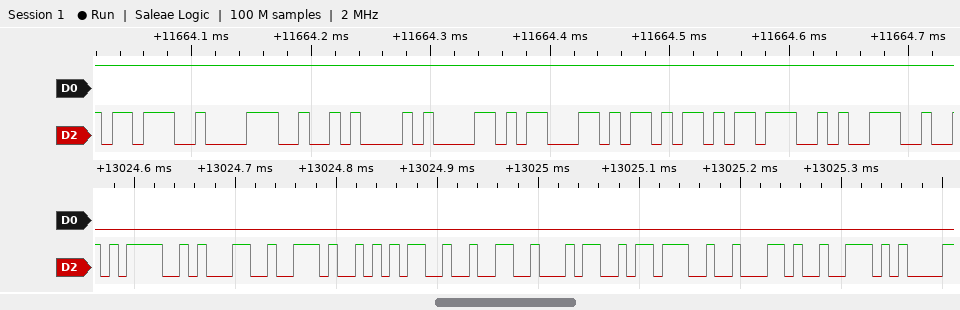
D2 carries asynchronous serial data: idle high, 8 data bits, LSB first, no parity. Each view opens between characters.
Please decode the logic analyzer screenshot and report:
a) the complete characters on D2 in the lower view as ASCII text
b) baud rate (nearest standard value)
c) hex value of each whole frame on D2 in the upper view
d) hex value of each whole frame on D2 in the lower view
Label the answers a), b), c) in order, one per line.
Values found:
a) "=1.524;br"
b) 115200 baud
c) 3B, 38, 0A, 61, 63, 6B, 3B, 39
d) 3D, 31, 2E, 35, 32, 34, 3B, 62, 72
